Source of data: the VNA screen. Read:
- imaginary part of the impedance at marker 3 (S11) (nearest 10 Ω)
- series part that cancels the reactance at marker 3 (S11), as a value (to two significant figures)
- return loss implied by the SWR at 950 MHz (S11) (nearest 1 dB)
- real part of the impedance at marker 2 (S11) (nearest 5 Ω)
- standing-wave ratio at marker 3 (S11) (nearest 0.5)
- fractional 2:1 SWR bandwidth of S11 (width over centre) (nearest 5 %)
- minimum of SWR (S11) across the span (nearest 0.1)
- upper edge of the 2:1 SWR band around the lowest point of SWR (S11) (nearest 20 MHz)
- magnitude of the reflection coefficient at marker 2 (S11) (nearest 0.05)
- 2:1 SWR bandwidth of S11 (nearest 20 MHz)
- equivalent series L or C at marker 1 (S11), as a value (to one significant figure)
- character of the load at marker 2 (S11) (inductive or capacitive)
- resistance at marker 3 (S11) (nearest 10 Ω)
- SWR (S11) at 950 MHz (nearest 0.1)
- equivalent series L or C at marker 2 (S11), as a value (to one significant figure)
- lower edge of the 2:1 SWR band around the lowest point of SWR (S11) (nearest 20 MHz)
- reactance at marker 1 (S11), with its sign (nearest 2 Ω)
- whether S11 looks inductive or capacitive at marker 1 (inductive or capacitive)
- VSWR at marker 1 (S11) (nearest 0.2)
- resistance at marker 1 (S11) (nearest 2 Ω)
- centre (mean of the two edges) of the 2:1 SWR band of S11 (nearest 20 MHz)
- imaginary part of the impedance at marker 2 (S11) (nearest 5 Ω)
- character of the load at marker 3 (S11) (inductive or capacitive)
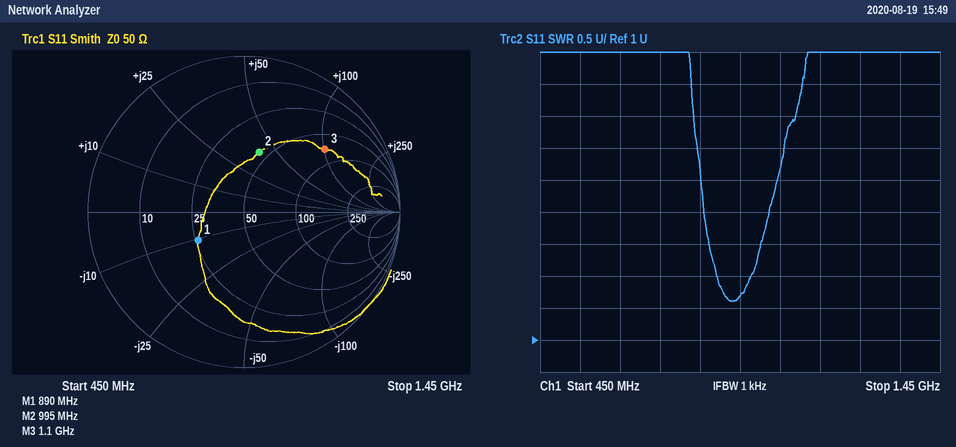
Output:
+100 Ω
1.4 pF
12 dB
45 Ω
5.0
10 %
1.6
980 MHz
0.40
80 MHz
20 pF
inductive
70 Ω
1.7
6 nH
900 MHz
-10 Ω
capacitive
2.0
26 Ω
940 MHz
+40 Ω
inductive
